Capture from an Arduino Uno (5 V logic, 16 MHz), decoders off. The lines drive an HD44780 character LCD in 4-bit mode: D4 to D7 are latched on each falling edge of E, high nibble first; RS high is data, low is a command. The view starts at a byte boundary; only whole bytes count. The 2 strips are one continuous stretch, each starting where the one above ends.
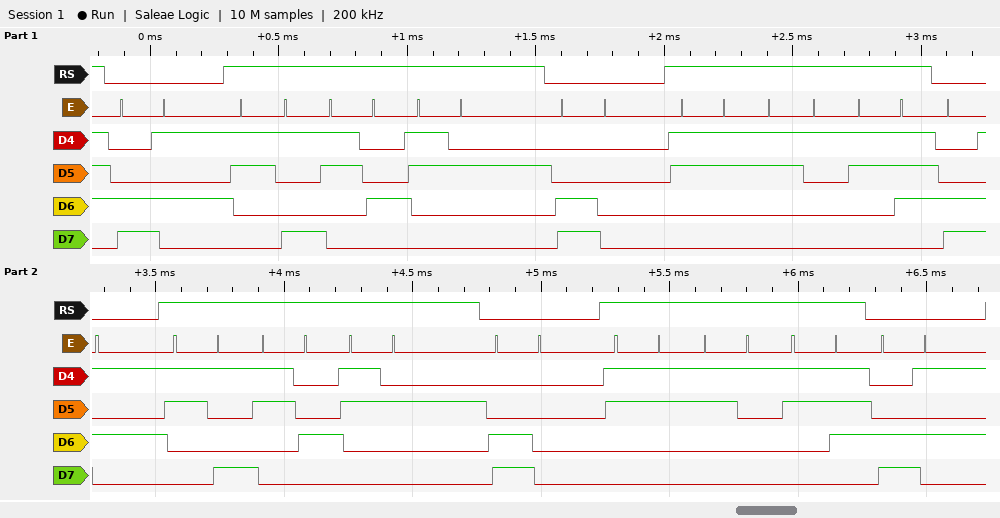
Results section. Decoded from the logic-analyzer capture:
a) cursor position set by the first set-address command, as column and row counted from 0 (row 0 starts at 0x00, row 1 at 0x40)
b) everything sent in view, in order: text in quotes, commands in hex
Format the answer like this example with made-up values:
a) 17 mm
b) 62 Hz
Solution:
a) column 5, row 1
b) 0xC5 "942" 0xC0 "317" 0xC5 "942" 0xC0 "317" 0xC5
